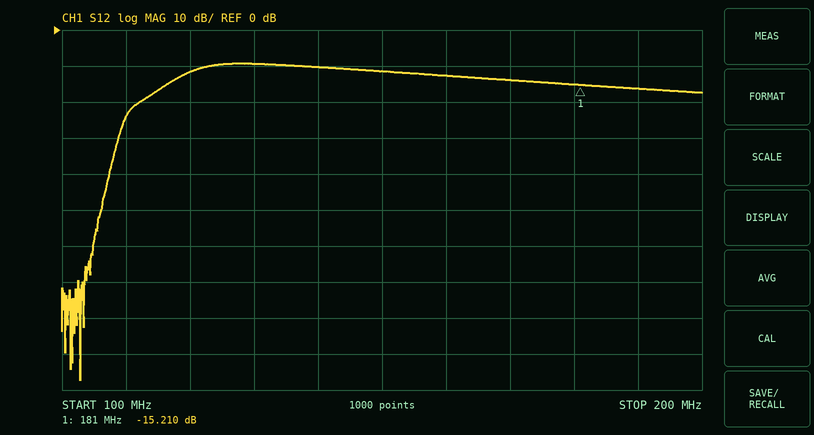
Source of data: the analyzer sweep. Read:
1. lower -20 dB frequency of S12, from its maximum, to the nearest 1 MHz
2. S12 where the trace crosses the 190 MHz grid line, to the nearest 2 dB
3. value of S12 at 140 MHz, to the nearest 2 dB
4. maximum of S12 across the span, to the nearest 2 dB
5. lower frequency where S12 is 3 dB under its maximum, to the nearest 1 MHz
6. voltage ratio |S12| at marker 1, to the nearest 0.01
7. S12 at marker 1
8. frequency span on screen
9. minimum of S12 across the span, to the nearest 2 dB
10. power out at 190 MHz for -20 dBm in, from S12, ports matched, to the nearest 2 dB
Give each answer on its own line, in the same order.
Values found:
109 MHz
-16 dB
-10 dB
-10 dB
119 MHz
0.17
-15.210 dB
100 MHz
-98 dB
-36 dBm
